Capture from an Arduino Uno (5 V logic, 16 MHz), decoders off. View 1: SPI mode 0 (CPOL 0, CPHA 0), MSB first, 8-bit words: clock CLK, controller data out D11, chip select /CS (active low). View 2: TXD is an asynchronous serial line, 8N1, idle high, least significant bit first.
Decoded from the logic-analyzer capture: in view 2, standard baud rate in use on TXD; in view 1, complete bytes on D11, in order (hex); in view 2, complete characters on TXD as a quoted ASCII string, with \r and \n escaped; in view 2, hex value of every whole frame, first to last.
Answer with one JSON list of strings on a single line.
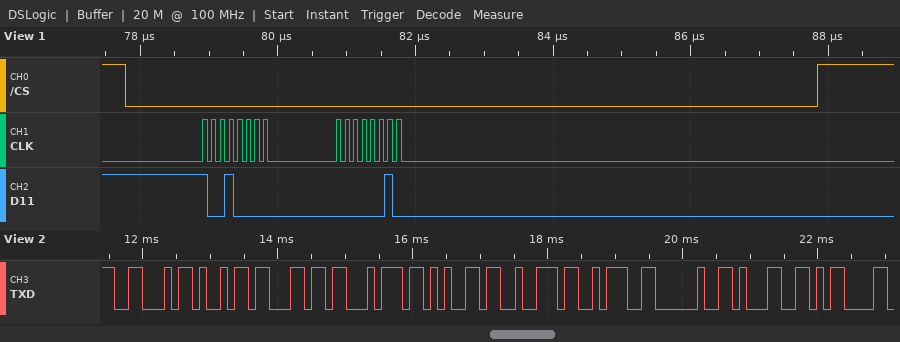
["9600 baud", "90 02", "\"Filter: 1\\r\"", "46 69 6C 74 65 72 3A 20 31 0D"]
